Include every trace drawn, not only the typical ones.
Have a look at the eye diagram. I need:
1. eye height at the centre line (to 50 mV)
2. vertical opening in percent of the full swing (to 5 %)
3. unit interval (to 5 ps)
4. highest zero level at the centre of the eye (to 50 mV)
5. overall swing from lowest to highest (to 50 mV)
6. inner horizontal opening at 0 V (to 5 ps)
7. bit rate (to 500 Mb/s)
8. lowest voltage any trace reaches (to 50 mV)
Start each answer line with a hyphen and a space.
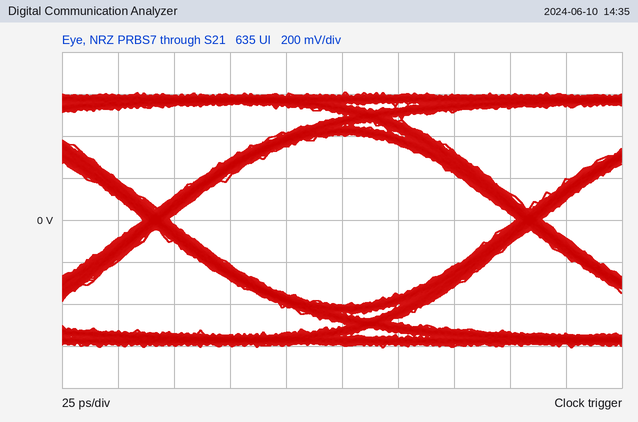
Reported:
- 800 mV
- 65 %
- 165 ps
- -400 mV
- 1.20 V
- 155 ps
- 6.0 Gb/s
- -600 mV
